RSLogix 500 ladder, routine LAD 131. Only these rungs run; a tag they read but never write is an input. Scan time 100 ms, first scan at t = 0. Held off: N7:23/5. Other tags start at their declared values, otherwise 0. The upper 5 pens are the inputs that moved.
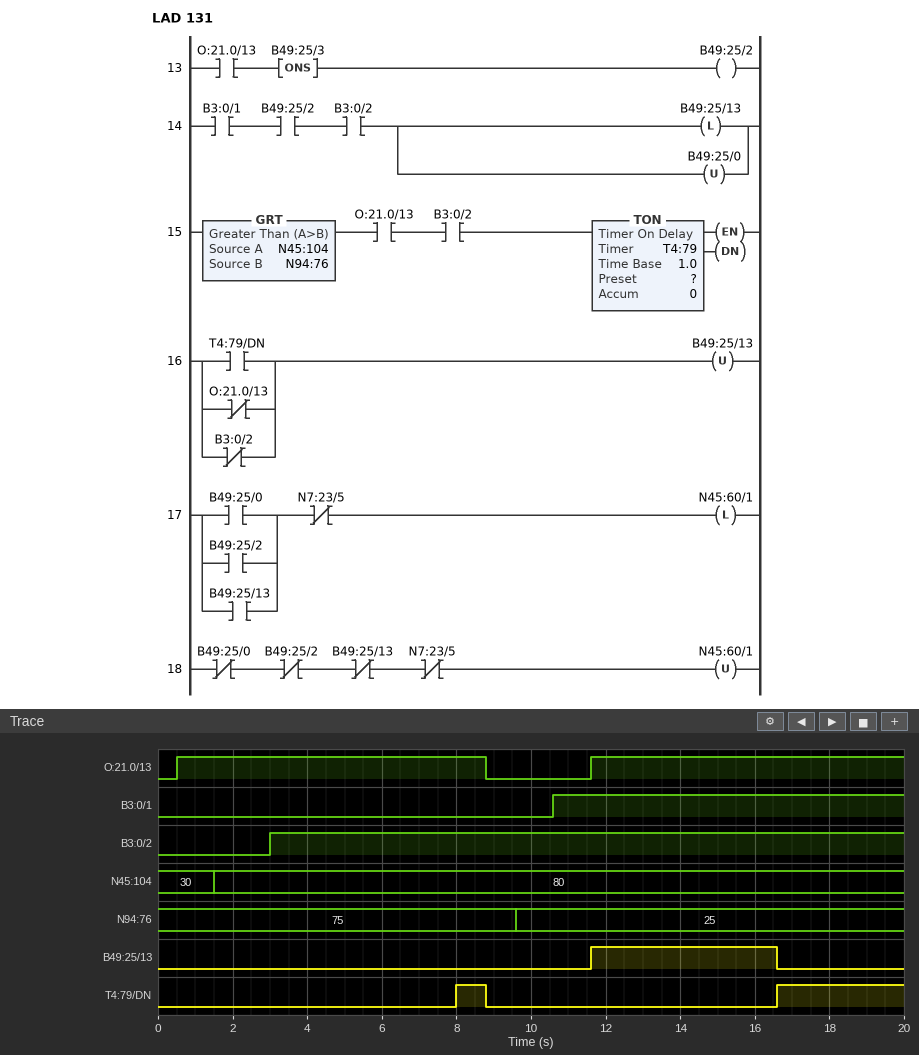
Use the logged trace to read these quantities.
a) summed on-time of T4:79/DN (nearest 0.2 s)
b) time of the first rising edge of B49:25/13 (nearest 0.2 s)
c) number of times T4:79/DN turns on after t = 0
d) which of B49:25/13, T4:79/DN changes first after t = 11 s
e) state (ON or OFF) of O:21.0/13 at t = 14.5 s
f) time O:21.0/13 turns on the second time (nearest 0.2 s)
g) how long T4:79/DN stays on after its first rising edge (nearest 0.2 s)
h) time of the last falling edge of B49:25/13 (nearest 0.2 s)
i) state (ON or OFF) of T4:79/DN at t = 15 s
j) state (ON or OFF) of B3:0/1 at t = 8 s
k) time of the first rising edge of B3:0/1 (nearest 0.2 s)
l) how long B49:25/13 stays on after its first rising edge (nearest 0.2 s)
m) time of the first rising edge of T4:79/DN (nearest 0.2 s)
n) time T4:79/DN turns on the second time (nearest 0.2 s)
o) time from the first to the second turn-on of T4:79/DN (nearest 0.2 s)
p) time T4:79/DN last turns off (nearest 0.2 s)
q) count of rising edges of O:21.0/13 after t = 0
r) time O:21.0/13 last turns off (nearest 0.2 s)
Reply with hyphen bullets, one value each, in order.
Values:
- 4.2 s
- 11.6 s
- 2
- B49:25/13
- ON
- 11.6 s
- 0.8 s
- 16.6 s
- OFF
- OFF
- 10.6 s
- 5.0 s
- 8.0 s
- 16.6 s
- 8.6 s
- 8.8 s
- 2
- 8.8 s
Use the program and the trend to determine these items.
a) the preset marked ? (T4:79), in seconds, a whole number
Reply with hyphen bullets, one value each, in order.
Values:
- 5 s
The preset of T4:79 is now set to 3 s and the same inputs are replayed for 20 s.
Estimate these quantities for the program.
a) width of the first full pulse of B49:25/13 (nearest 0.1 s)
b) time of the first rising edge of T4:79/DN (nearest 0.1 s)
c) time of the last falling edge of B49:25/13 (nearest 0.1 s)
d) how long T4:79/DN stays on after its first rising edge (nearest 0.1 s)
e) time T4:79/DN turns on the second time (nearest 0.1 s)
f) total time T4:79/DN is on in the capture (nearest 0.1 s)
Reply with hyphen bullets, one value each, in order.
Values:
- 3.0 s
- 6.0 s
- 14.6 s
- 2.8 s
- 14.6 s
- 8.2 s
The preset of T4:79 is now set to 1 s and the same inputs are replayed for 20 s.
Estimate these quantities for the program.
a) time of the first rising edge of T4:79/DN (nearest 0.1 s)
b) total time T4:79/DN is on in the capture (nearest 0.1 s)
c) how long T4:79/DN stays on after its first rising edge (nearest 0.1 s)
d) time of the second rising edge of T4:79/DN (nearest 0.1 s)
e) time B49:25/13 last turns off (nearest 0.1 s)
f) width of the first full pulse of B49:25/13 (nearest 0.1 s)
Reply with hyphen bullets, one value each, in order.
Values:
- 4.0 s
- 12.2 s
- 4.8 s
- 12.6 s
- 12.6 s
- 1.0 s
